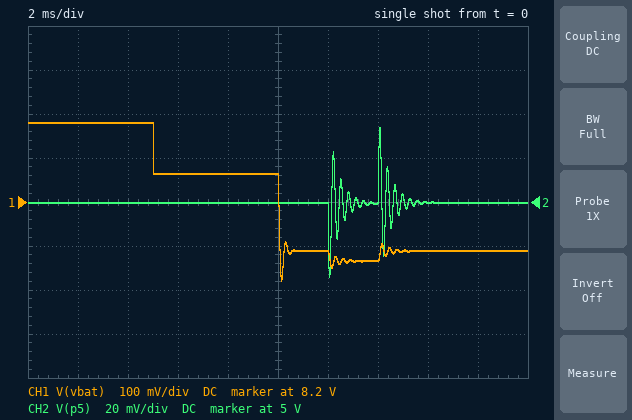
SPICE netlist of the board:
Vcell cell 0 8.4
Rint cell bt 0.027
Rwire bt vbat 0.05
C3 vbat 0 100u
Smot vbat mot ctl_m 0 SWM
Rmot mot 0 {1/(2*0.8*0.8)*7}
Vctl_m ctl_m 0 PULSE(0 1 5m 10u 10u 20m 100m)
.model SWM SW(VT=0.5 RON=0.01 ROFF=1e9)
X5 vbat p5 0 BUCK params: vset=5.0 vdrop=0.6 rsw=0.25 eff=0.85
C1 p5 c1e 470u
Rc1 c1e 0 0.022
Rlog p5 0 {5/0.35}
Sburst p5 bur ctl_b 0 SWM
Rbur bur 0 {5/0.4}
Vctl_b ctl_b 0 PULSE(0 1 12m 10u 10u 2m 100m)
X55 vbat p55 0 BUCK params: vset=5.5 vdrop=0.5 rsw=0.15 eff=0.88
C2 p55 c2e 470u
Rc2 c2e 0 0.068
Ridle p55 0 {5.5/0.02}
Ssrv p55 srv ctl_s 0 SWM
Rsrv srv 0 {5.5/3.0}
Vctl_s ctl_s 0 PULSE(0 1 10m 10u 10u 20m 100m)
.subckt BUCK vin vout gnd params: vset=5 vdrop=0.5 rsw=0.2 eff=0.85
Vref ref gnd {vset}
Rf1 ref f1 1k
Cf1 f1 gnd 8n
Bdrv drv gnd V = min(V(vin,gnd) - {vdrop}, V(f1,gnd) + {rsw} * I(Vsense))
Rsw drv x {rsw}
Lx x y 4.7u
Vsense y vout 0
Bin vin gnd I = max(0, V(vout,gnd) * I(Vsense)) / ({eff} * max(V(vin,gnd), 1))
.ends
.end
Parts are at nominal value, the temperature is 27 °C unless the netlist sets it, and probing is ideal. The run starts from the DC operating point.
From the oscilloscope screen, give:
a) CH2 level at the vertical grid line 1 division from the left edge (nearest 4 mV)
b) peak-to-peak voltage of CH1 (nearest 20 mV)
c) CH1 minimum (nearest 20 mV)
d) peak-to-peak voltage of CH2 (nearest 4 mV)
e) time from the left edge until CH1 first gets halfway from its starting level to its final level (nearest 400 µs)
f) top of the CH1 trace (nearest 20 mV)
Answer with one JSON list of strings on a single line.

["5.000 V", "360 mV", "8.02 V", "68 mV", "10.0 ms", "8.38 V"]
